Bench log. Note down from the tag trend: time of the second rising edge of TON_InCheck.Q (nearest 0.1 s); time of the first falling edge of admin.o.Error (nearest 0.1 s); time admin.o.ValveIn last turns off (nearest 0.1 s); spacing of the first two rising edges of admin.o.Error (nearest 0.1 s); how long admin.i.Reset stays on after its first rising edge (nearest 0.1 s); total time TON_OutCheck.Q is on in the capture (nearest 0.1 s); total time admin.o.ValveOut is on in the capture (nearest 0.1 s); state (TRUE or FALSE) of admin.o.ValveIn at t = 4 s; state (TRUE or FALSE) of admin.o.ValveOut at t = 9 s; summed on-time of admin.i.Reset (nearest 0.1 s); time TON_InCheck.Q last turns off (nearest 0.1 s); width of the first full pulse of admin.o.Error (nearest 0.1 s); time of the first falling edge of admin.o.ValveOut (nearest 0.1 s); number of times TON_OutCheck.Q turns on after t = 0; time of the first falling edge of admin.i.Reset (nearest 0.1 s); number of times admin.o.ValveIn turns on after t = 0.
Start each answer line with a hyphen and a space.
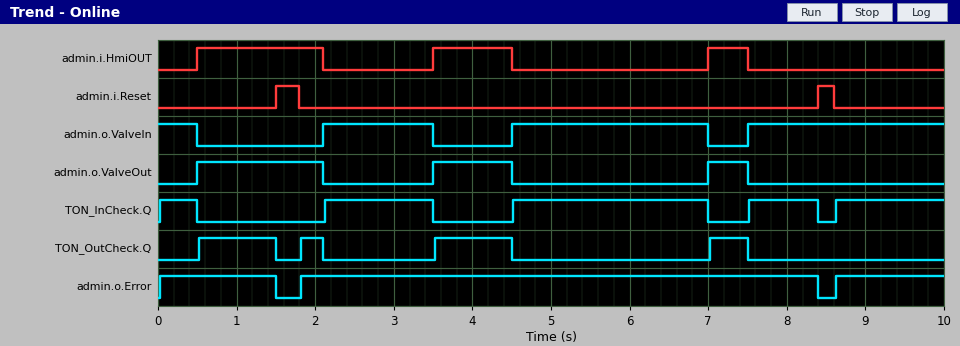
- 2.1 s
- 1.5 s
- 7.0 s
- 1.8 s
- 0.3 s
- 2.7 s
- 3.1 s
- FALSE
- FALSE
- 0.5 s
- 8.4 s
- 1.5 s
- 2.1 s
- 4
- 1.8 s
- 3
